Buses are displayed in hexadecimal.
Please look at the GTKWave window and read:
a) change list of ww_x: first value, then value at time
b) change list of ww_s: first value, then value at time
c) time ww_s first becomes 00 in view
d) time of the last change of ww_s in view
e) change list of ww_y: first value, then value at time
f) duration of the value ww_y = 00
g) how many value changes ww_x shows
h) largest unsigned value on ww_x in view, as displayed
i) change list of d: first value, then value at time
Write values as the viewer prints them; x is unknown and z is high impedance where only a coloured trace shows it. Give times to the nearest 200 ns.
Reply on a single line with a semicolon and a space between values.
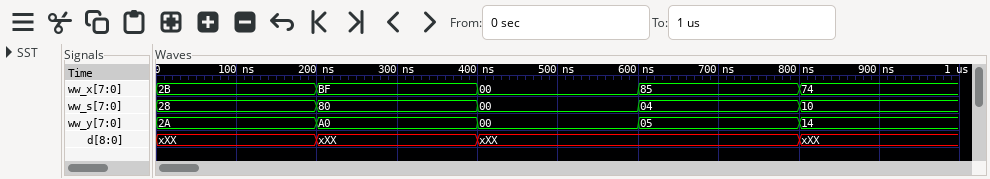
2B, BF at 200 ns, 00 at 400 ns, 85 at 600 ns, 74 at 800 ns; 28, 80 at 200 ns, 00 at 400 ns, 04 at 600 ns, 10 at 800 ns; 400 ns; 800 ns; 2A, A0 at 200 ns, 00 at 400 ns, 05 at 600 ns, 14 at 800 ns; 200 ns; 4; BF; xXX, xXX at 200 ns, xXX at 400 ns, xXX at 800 ns
